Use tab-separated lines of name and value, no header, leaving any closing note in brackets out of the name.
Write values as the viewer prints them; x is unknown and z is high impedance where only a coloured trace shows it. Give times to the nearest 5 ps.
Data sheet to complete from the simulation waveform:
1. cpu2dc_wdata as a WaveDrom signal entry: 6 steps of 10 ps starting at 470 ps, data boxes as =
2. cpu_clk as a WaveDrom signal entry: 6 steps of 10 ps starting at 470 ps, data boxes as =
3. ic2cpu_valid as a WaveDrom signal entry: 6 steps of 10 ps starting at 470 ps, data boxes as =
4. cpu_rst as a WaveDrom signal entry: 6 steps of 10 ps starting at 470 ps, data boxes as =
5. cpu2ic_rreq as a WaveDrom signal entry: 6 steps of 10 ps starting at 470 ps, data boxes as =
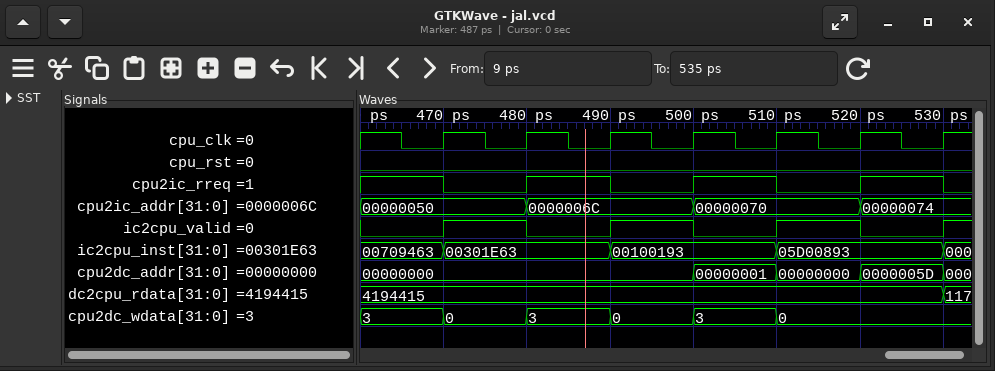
cpu2dc_wdata as a WaveDrom signal entry: 6 steps of 10 ps starting at 470 ps, data boxes as =	{name: 'cpu2dc_wdata', wave: '=====.', data: '0 3 0 3 0'}
cpu_clk as a WaveDrom signal entry: 6 steps of 10 ps starting at 470 ps, data boxes as =	{name: 'cpu_clk', wave: 'p.....'}
ic2cpu_valid as a WaveDrom signal entry: 6 steps of 10 ps starting at 470 ps, data boxes as =	{name: 'ic2cpu_valid', wave: '101010'}
cpu_rst as a WaveDrom signal entry: 6 steps of 10 ps starting at 470 ps, data boxes as =	{name: 'cpu_rst', wave: '0.....'}
cpu2ic_rreq as a WaveDrom signal entry: 6 steps of 10 ps starting at 470 ps, data boxes as =	{name: 'cpu2ic_rreq', wave: '010101'}
